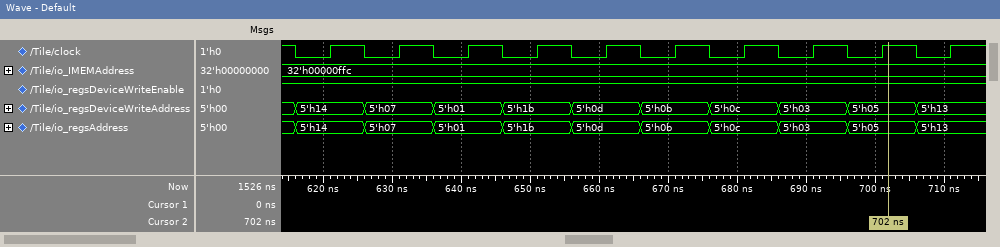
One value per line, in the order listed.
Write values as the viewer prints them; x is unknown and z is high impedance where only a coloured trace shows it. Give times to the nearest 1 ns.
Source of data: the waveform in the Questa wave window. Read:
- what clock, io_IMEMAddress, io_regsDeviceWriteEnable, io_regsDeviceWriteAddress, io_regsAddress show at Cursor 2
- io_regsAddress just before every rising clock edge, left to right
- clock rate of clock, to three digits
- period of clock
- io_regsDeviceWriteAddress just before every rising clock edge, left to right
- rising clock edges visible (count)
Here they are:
clock=1, io_IMEMAddress=32'h00000ffc, io_regsDeviceWriteEnable=1, io_regsDeviceWriteAddress=5'h05, io_regsAddress=5'h05
5'h14, 5'h07, 5'h01, 5'h1b, 5'h0d, 5'h0b, 5'h0c, 5'h03, 5'h05, 5'h13
100 MHz
10 ns
5'h14, 5'h07, 5'h01, 5'h1b, 5'h0d, 5'h0b, 5'h0c, 5'h03, 5'h05, 5'h13
10
